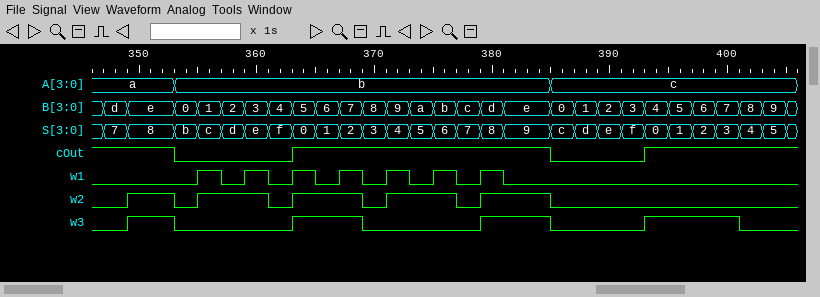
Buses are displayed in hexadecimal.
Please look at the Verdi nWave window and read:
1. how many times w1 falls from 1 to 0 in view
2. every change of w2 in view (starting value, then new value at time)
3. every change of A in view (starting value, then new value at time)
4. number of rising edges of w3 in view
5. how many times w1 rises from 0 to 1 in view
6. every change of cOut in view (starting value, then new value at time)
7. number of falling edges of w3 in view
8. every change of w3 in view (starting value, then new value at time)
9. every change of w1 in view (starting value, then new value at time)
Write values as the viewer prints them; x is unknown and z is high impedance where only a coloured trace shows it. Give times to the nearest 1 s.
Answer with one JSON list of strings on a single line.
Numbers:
["7", "0, 1 at 349 s, 0 at 353 s, 1 at 355 s, 0 at 361 s, 1 at 363 s, 0 at 369 s, 1 at 371 s, 0 at 377 s, 1 at 379 s, 0 at 385 s", "a, b at 353 s, c at 385 s", "4", "7", "1, 0 at 353 s, 1 at 363 s, 0 at 385 s, 1 at 393 s", "4", "0, 1 at 349 s, 0 at 353 s, 1 at 363 s, 0 at 369 s, 1 at 379 s, 0 at 385 s, 1 at 393 s, 0 at 401 s", "0, 1 at 355 s, 0 at 357 s, 1 at 359 s, 0 at 361 s, 1 at 363 s, 0 at 365 s, 1 at 367 s, 0 at 369 s, 1 at 371 s, 0 at 373 s, 1 at 375 s, 0 at 377 s, 1 at 379 s, 0 at 381 s"]
